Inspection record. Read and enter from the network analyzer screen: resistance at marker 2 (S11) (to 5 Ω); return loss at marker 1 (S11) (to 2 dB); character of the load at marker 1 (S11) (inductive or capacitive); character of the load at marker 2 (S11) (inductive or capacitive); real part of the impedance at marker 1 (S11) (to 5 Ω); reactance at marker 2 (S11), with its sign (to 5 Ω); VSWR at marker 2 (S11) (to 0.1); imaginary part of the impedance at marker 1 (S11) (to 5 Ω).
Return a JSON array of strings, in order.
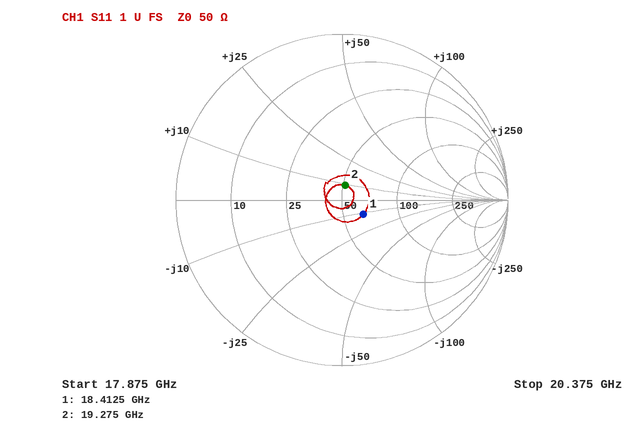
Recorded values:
["50 Ω", "16 dB", "capacitive", "inductive", "65 Ω", "+10 Ω", "1.2", "-10 Ω"]
